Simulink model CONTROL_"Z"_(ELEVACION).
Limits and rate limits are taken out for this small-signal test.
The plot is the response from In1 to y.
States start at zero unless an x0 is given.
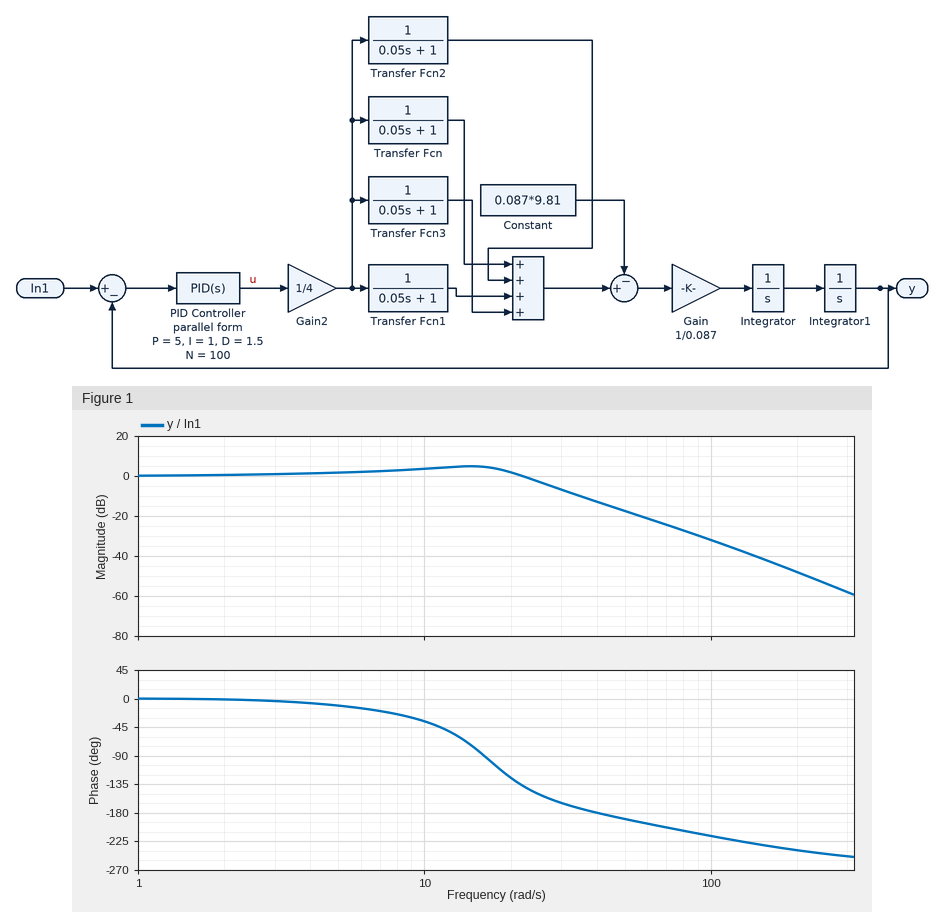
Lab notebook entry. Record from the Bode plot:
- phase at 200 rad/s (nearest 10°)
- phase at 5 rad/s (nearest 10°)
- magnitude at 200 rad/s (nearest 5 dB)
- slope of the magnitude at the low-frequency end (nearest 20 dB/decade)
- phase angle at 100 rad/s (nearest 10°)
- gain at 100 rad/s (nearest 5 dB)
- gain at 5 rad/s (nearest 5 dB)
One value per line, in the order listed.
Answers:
-240°
-10°
-50 dB
0 dB/decade
-220°
-30 dB
0 dB
